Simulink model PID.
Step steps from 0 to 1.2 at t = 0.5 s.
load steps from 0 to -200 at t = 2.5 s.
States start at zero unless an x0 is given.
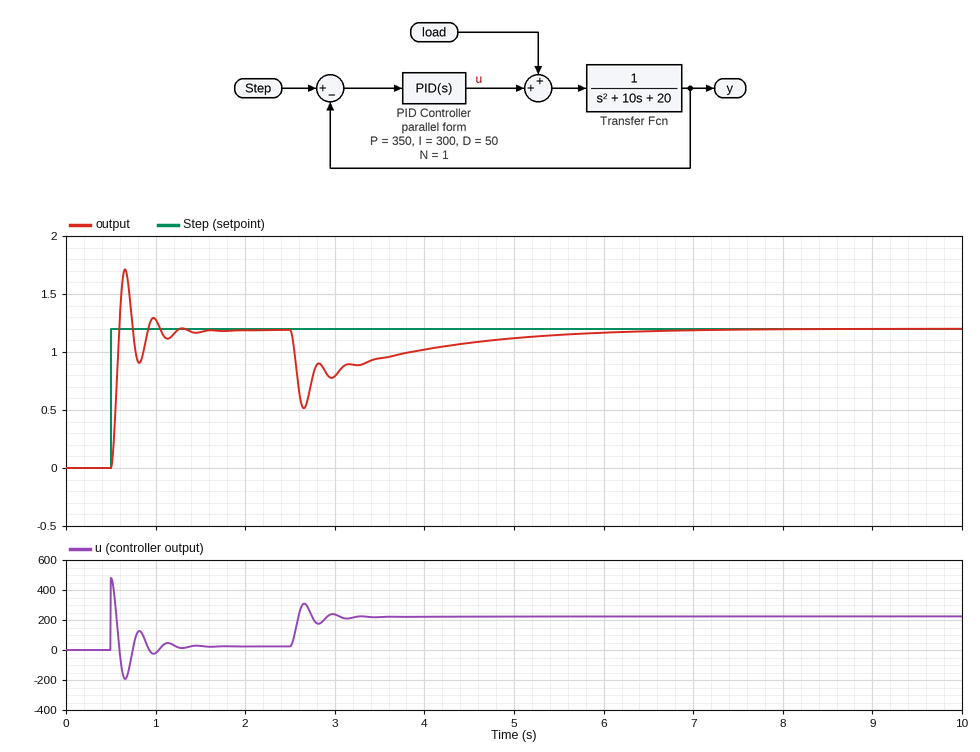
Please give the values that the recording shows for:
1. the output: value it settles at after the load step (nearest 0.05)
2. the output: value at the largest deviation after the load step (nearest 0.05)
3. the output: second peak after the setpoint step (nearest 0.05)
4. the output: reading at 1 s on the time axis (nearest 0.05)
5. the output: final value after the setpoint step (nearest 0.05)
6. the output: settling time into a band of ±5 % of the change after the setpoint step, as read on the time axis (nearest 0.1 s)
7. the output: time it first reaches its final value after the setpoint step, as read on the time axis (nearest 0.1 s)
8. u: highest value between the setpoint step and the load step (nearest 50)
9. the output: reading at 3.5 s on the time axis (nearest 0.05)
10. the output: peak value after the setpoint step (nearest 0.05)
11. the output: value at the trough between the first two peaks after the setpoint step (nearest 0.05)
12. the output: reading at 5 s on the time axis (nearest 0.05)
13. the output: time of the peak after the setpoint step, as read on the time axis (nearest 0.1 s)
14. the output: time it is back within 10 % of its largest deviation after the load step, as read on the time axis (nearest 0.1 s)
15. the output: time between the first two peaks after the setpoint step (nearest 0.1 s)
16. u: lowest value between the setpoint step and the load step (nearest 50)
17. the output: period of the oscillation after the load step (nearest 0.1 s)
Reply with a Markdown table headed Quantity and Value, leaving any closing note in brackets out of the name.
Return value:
| Quantity | Value |
|---|---|
| the output: value it settles at after the load step | 1.20 |
| the output: value at the largest deviation after the load step | 0.50 |
| the output: second peak after the setpoint step | 1.30 |
| the output: reading at 1 s on the time axis | 1.30 |
| the output: final value after the setpoint step | 1.20 |
| the output: settling time into a band of ±5 % of the change after the setpoint step, as read on the time axis | 1.2 s |
| the output: time it first reaches its final value after the setpoint step, as read on the time axis | 0.6 s |
| u: highest value between the setpoint step and the load step | 500 |
| the output: reading at 3.5 s on the time axis | 0.95 |
| the output: peak value after the setpoint step | 1.70 |
| the output: value at the trough between the first two peaks after the setpoint step | 0.90 |
| the output: reading at 5 s on the time axis | 1.10 |
| the output: time of the peak after the setpoint step, as read on the time axis | 0.7 s |
| the output: time it is back within 10 % of its largest deviation after the load step, as read on the time axis | 5.2 s |
| the output: time between the first two peaks after the setpoint step | 0.3 s |
| u: lowest value between the setpoint step and the load step | -200 |
| the output: period of the oscillation after the load step | 0.3 s |
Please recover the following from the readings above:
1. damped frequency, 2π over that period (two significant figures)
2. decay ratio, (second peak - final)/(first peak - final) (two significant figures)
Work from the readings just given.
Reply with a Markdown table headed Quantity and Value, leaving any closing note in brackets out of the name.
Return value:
| Quantity | Value |
|---|---|
| damped frequency, 2π over that period | 21 rad/s |
| decay ratio, (second peak - final)/(first peak - final) | 0.20 |
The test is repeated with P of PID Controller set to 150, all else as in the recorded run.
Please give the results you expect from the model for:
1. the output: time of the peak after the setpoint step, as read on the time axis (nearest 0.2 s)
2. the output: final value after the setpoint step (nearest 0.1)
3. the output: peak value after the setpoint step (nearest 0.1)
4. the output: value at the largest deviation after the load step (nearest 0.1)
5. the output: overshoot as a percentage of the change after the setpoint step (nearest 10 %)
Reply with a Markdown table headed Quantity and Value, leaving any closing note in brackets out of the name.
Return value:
| Quantity | Value |
|---|---|
| the output: time of the peak after the setpoint step, as read on the time axis | 0.8 s |
| the output: final value after the setpoint step | 1.2 |
| the output: peak value after the setpoint step | 1.6 |
| the output: value at the largest deviation after the load step | 0.1 |
| the output: overshoot as a percentage of the change after the setpoint step | 30 % |
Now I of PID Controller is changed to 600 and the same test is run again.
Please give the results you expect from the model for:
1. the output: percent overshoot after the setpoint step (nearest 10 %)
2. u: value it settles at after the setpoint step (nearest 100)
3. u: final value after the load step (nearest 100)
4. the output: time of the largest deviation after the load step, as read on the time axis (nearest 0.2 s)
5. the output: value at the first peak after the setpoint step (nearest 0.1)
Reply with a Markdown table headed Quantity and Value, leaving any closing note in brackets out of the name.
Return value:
| Quantity | Value |
|---|---|
| the output: percent overshoot after the setpoint step | 50 % |
| u: value it settles at after the setpoint step | 0 |
| u: final value after the load step | 200 |
| the output: time of the largest deviation after the load step, as read on the time axis | 2.6 s |
| the output: value at the first peak after the setpoint step | 1.8 |
